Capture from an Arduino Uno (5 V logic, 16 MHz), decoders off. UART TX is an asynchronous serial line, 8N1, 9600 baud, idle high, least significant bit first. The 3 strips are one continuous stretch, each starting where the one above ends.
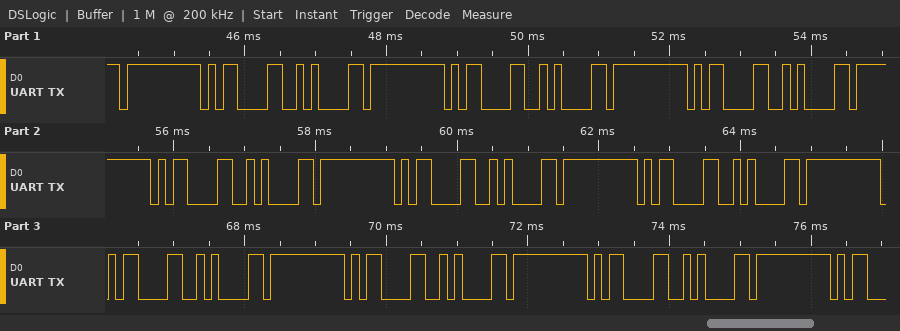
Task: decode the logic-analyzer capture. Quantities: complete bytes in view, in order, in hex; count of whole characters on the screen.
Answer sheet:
FF 0D 0A FF 0D 0A FF 0D 0A FF 0D 0A FF 0D 0A FF 0D 0A FF 0D 0A FF 0D 0A FF 0D 0A FF
28
